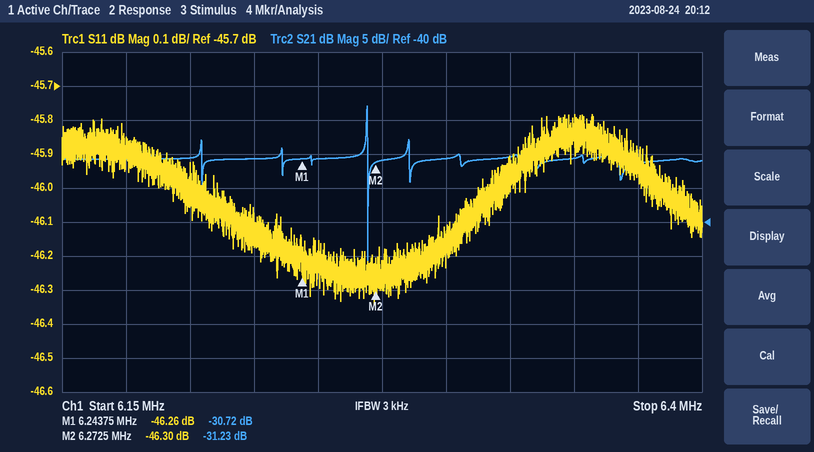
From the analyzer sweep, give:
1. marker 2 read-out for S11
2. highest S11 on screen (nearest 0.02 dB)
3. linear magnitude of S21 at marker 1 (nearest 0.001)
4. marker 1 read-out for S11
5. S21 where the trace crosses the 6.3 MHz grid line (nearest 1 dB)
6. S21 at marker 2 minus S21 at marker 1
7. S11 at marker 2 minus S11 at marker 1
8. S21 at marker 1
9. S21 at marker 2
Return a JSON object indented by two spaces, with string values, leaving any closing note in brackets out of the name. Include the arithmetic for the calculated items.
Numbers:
{
  "marker 2 read-out for S11": "-46.30 dB",
  "highest S11 on screen": "-45.78 dB",
  "linear magnitude of S21 at marker 1": "10^(-30.72/20) ≈ 0.029",
  "marker 1 read-out for S11": "-46.26 dB",
  "S21 where the trace crosses the 6.3 MHz grid line": "-31 dB",
  "S21 at marker 2 minus S21 at marker 1": "-31.23 − (-30.72) = -0.51 dB",
  "S11 at marker 2 minus S11 at marker 1": "-46.3 − (-46.26) = -0.04 dB",
  "S21 at marker 1": "-30.72 dB",
  "S21 at marker 2": "-31.23 dB"
}
